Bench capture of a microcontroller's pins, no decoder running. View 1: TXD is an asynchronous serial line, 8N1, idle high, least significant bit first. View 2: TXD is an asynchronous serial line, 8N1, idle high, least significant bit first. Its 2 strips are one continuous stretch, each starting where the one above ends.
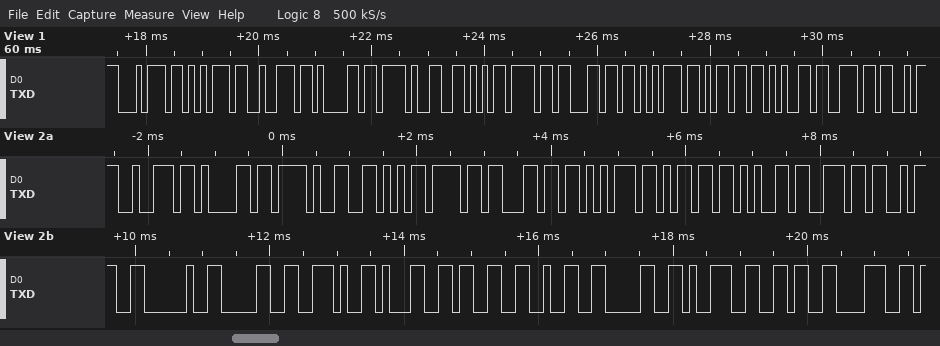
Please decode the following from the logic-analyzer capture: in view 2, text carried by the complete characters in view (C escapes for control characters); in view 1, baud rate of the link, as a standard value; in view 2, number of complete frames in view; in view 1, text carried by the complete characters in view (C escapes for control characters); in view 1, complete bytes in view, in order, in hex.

"ra/Volumen: 0.1320968"
9600 baud
21
"tura/Volumen"
74 75 72 61 2F 56 6F 6C 75 6D 65 6E
